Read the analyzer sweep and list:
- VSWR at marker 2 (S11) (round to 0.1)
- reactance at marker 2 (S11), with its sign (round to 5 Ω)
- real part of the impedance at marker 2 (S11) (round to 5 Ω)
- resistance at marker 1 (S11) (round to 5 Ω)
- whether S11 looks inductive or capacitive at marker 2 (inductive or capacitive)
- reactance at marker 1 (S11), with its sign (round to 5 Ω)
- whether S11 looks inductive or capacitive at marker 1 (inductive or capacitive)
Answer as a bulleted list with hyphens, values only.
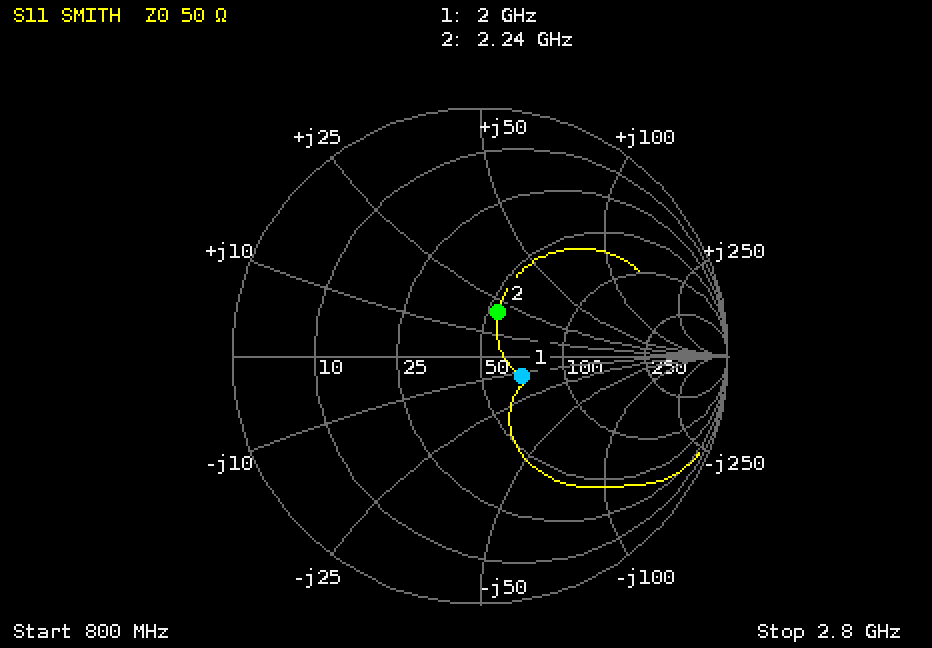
- 1.5
- +20 Ω
- 55 Ω
- 70 Ω
- inductive
- -10 Ω
- capacitive
